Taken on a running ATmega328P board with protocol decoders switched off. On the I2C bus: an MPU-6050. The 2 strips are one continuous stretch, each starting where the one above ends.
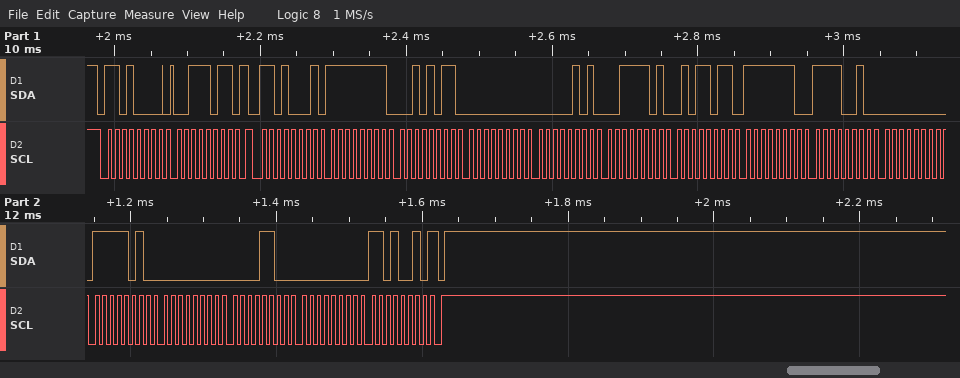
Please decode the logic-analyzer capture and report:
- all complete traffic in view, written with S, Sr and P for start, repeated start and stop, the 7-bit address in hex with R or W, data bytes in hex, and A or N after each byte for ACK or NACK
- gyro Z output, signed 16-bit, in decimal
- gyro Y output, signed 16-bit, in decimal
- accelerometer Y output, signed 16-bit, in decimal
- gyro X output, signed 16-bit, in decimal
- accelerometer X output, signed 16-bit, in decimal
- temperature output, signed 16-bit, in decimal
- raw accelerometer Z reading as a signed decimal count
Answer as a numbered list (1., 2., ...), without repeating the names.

1. S 68W A 3B A Sr 68R A FF A 2B A 00 A 05 A 3D A 5B A FE A F2 A 00 A FA A 00 A 0C A 00 A D2 N P
2. 210
3. 12
4. 5
5. 250
6. -213
7. -270
8. 15707
